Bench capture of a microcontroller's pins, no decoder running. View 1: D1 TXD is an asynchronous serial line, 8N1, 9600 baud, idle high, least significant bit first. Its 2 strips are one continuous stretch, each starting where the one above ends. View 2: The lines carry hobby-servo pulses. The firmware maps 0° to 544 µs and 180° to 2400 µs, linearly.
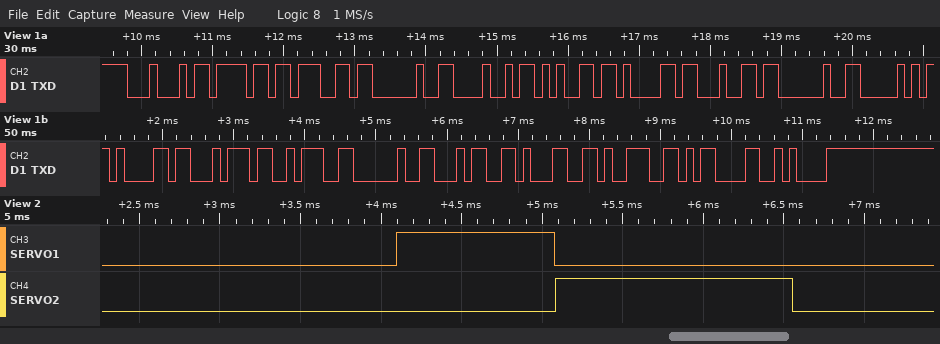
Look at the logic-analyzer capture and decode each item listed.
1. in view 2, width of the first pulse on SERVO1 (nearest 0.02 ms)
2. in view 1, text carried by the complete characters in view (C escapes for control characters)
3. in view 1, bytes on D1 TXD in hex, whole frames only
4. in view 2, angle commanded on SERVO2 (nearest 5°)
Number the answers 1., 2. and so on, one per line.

1. 0.98 ms
2. "Dog Head Pat: 419\r\n"
3. 0x44 0x6F 0x67 0x20 0x48 0x65 0x61 0x64 0x20 0x50 0x61 0x74 0x3A 0x20 0x34 0x31 0x39 0x0D 0x0A
4. 90°
